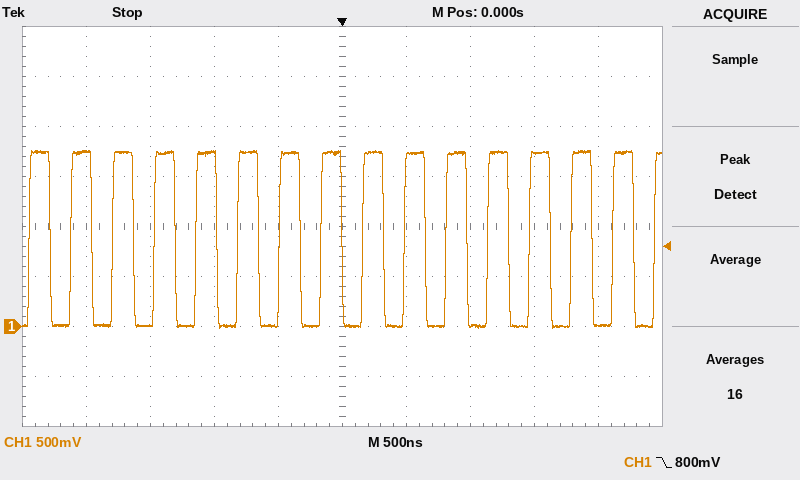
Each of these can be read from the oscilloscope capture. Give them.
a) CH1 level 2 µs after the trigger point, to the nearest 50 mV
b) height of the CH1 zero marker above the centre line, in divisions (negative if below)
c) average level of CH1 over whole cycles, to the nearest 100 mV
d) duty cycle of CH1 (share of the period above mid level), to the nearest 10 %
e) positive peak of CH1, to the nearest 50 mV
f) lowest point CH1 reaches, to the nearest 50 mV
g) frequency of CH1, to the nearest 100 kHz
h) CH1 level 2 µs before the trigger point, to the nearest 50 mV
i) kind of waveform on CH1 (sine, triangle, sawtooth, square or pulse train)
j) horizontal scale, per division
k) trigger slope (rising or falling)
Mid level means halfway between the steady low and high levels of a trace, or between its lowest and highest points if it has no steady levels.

0 mV
-2.0 div
900 mV
50 %
1.75 V
0 mV
3.1 MHz
1.75 V
square
500 ns
falling
